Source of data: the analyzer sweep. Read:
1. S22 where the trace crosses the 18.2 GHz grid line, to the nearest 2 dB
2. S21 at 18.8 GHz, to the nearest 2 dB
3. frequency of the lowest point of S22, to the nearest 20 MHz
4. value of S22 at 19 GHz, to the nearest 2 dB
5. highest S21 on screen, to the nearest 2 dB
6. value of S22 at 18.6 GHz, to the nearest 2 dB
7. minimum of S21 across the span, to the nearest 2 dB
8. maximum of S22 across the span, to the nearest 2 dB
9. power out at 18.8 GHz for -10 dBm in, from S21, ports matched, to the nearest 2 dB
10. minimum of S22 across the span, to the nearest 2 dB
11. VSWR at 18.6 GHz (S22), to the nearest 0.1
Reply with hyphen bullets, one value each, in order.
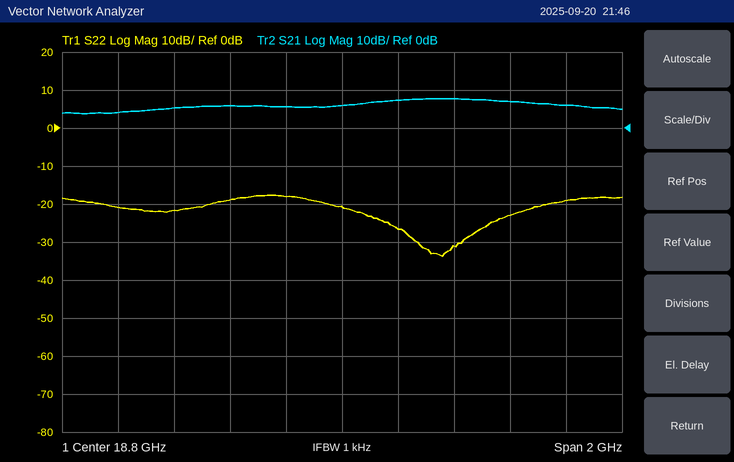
- -22 dB
- 6 dB
- 19.16 GHz
- -26 dB
- 8 dB
- -18 dB
- 4 dB
- -18 dB
- -4 dBm
- -34 dB
- 1.3
